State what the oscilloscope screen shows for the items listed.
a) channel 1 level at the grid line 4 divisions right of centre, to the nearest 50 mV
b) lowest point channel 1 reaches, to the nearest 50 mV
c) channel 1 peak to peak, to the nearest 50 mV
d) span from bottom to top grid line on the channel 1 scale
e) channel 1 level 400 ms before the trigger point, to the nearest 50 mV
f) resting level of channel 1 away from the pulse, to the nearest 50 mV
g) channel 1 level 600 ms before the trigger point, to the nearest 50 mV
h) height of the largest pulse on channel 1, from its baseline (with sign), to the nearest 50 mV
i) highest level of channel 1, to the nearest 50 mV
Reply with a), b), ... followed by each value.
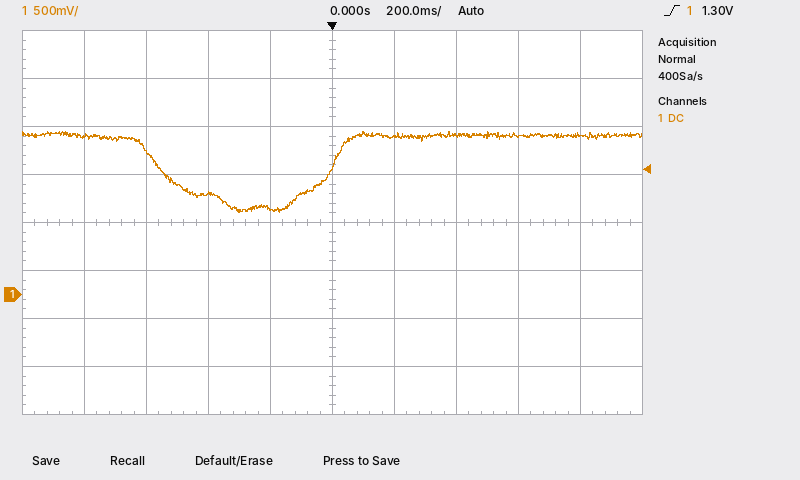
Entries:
a) 1.65 V
b) 850 mV
c) 850 mV
d) 4 V
e) 1.05 V
f) 1.65 V
g) 1.50 V
h) -800 mV
i) 1.70 V
